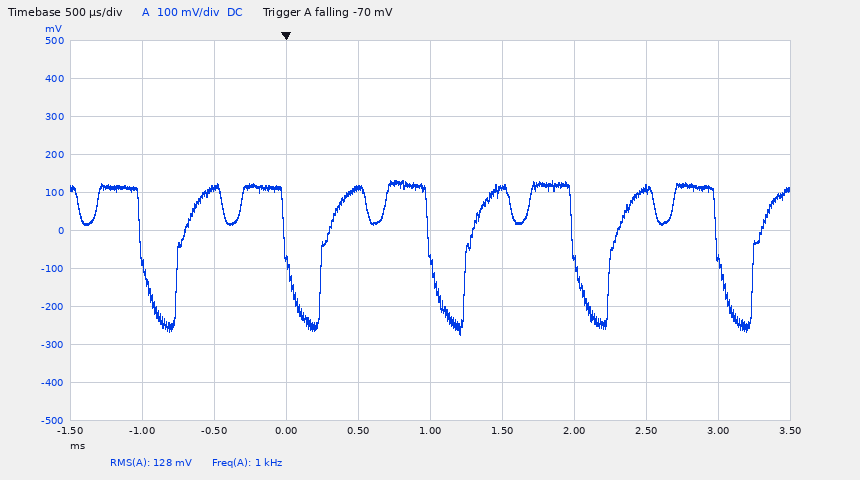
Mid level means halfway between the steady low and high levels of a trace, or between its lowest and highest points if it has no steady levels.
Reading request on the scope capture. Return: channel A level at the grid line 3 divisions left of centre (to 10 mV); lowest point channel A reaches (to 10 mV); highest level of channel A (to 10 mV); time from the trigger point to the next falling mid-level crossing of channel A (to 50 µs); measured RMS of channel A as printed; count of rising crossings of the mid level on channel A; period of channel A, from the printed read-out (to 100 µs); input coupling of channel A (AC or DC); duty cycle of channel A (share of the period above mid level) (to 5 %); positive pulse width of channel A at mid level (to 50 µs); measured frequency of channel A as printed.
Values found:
110 mV
-270 mV
130 mV
1.00 ms
128 mV
5
1.0 ms
DC
75 %
750 µs
1 kHz
